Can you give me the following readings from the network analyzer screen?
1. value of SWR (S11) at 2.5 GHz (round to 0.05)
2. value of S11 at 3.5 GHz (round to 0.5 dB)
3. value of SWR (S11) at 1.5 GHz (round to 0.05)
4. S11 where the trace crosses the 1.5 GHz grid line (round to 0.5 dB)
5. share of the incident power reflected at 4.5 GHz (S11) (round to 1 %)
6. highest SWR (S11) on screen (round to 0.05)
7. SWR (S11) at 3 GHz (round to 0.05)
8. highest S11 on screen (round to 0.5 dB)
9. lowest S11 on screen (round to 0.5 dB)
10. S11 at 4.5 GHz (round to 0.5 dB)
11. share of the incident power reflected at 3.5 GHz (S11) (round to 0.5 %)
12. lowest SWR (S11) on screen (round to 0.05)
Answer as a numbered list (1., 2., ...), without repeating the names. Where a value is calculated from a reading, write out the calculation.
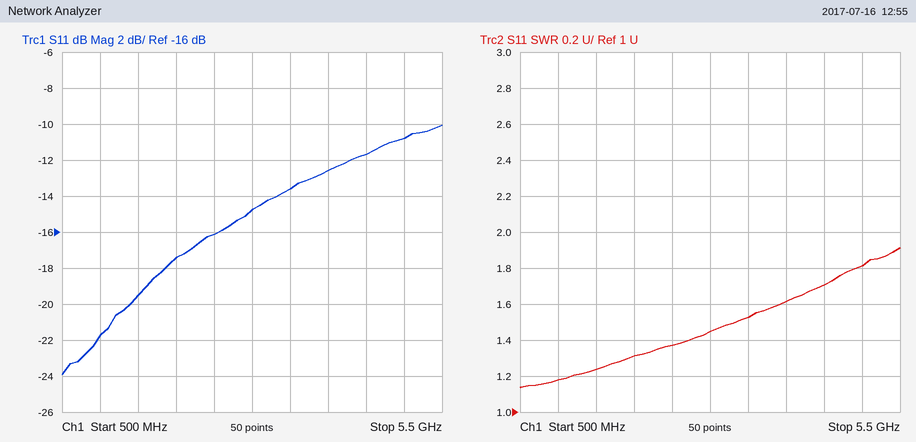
1. 1.35
2. -13.5 dB
3. 1.25
4. -19.5 dB
5. 10^(-11.5/10) ≈ 7 %
6. 1.90
7. 1.45
8. -10.0 dB
9. -24.0 dB
10. -11.5 dB
11. 10^(-13.5/10) ≈ 4.5 %
12. 1.15
